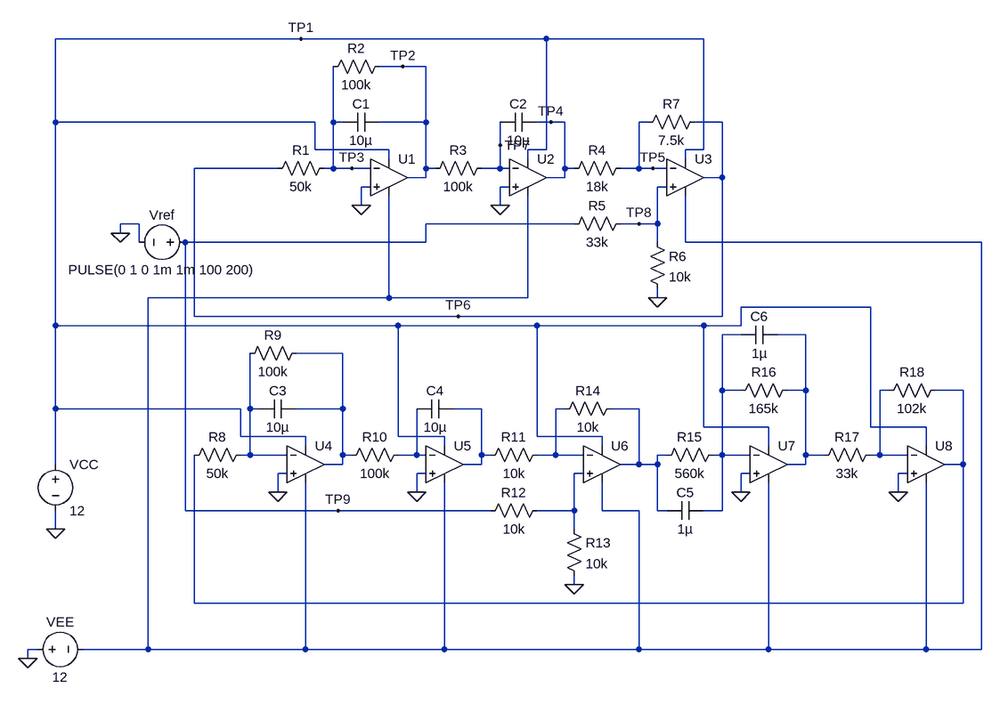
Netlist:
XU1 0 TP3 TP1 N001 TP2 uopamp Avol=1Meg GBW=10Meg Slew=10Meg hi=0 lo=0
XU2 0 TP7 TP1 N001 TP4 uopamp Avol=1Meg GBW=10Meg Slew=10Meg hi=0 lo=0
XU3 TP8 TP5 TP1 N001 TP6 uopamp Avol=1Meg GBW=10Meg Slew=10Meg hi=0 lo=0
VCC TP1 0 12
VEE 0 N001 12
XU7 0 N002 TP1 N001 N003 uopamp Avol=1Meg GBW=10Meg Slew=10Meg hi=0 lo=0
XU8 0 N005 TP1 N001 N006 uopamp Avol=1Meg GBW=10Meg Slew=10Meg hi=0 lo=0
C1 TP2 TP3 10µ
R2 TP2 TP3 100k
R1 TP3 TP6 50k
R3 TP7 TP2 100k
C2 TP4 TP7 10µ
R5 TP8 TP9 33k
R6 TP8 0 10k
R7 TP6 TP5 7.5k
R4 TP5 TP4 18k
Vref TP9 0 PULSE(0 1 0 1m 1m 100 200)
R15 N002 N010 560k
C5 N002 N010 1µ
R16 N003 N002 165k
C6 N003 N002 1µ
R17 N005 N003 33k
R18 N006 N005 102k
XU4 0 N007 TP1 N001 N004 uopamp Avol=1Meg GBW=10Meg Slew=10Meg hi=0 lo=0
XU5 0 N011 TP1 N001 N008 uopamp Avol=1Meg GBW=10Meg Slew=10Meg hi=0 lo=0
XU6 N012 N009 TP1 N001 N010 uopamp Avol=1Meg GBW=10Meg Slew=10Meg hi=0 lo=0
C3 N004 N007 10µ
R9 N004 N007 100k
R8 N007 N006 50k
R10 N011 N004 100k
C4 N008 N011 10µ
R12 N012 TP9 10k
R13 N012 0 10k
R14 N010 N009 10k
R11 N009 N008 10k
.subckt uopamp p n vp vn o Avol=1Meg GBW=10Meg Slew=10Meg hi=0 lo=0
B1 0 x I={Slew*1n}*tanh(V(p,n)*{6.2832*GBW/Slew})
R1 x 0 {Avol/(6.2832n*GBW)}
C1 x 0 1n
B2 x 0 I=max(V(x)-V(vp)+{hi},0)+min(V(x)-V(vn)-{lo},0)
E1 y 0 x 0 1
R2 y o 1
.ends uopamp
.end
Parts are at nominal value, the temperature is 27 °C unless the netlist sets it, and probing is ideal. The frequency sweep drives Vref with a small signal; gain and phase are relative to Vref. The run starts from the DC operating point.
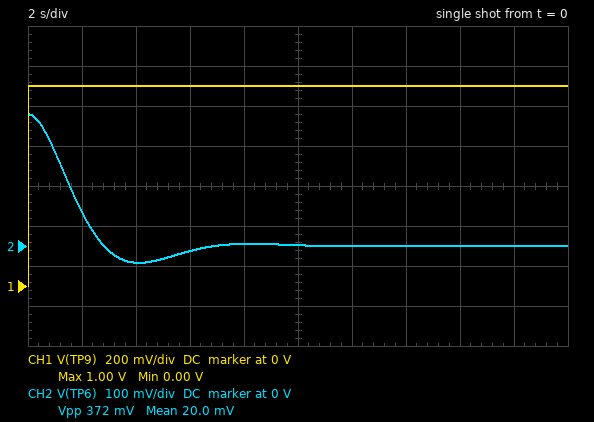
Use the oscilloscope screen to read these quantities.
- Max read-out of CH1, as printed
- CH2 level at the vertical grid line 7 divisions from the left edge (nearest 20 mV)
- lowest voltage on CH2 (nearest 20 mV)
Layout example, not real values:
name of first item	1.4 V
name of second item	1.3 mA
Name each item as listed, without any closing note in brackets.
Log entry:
Max read-out of CH1, as printed	1.00 V
CH2 level at the vertical grid line 7 divisions from the left edge	0 V
lowest voltage on CH2	-40 mV
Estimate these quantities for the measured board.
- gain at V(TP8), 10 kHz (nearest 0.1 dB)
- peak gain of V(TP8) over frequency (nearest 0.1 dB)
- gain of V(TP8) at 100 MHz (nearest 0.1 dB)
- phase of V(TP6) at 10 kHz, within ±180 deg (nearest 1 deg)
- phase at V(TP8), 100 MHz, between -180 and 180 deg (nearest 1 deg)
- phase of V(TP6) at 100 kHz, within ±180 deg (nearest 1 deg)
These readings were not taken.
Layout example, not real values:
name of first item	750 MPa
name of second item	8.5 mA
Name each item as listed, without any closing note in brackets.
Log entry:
gain at V(TP8), 10 kHz	-12.7 dB
peak gain of V(TP8) over frequency	-12.7 dB
gain of V(TP8) at 100 MHz	-12.7 dB
phase of V(TP6) at 10 kHz, within ±180 deg	0 deg
phase at V(TP8), 100 MHz, between -180 and 180 deg	0 deg
phase of V(TP6) at 100 kHz, within ±180 deg	-1 deg
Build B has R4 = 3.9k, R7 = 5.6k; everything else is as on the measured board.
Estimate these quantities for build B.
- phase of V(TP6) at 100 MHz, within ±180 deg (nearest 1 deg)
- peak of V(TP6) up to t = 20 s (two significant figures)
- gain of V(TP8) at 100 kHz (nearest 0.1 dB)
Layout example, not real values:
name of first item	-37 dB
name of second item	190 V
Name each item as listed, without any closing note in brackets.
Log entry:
phase of V(TP6) at 100 MHz, within ±180 deg	-88 deg
peak of V(TP6) up to t = 20 s	570 mV
gain of V(TP8) at 100 kHz	-12.7 dB
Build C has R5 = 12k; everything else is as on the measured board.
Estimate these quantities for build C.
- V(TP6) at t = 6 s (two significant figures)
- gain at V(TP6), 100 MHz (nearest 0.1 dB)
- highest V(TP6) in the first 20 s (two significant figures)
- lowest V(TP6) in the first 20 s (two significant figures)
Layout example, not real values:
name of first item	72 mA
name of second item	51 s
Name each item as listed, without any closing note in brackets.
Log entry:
V(TP6) at t = 6 s	-25 mV
gain at V(TP6), 100 MHz	-26.9 dB
highest V(TP6) in the first 20 s	640 mV
lowest V(TP6) in the first 20 s	-82 mV
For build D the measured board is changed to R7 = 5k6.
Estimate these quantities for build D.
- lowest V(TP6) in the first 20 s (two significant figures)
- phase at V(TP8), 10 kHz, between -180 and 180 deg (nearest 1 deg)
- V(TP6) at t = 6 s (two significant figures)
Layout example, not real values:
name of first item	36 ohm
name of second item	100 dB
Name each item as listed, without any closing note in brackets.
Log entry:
lowest V(TP6) in the first 20 s	-23 mV
phase at V(TP8), 10 kHz, between -180 and 180 deg	0 deg
V(TP6) at t = 6 s	-19 mV
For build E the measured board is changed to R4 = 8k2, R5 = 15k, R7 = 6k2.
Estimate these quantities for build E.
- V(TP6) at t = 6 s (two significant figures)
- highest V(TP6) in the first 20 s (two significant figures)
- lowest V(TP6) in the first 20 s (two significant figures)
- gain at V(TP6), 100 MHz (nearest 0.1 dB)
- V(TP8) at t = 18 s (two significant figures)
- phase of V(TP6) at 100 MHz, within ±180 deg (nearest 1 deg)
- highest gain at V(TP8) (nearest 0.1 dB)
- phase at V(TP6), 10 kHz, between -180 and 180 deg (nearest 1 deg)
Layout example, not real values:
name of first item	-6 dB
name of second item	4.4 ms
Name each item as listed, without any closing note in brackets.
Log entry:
V(TP6) at t = 6 s	38 mV
highest V(TP6) in the first 20 s	700 mV
lowest V(TP6) in the first 20 s	-170 mV
gain at V(TP6), 100 MHz	-28.0 dB
V(TP8) at t = 18 s	400 mV
phase of V(TP6) at 100 MHz, within ±180 deg	-87 deg
highest gain at V(TP8)	-8.0 dB
phase at V(TP6), 10 kHz, between -180 and 180 deg	0 deg
